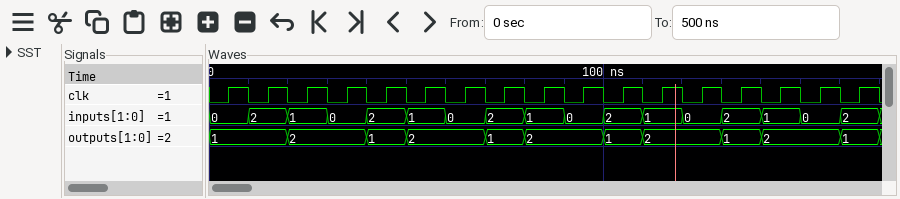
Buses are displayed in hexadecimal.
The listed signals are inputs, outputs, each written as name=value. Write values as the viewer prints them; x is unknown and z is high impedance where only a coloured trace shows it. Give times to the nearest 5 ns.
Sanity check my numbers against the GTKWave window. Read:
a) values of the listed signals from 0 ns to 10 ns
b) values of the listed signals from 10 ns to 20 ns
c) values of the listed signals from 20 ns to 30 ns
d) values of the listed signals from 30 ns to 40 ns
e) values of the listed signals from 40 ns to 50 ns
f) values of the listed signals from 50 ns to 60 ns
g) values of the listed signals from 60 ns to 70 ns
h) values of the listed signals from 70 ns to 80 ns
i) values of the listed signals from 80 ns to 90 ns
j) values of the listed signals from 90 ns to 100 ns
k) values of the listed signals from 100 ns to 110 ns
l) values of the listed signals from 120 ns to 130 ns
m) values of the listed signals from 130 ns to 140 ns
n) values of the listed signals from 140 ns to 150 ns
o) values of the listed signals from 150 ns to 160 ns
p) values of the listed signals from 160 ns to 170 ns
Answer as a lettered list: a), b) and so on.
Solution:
a) inputs=0, outputs=1
b) inputs=2, outputs=1
c) inputs=1, outputs=2
d) inputs=0, outputs=2
e) inputs=2, outputs=1
f) inputs=1, outputs=2
g) inputs=0, outputs=2
h) inputs=2, outputs=1
i) inputs=1, outputs=2
j) inputs=0, outputs=2
k) inputs=2, outputs=1
l) inputs=0, outputs=2
m) inputs=2, outputs=1
n) inputs=1, outputs=2
o) inputs=0, outputs=2
p) inputs=2, outputs=1
